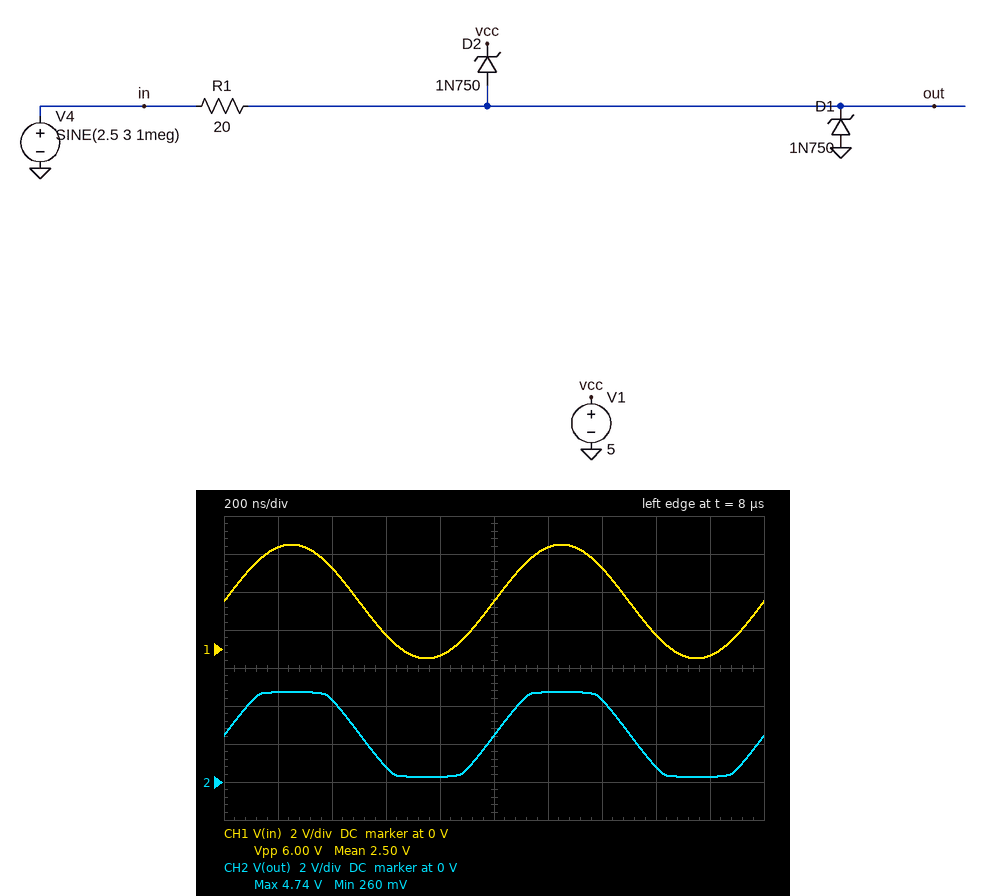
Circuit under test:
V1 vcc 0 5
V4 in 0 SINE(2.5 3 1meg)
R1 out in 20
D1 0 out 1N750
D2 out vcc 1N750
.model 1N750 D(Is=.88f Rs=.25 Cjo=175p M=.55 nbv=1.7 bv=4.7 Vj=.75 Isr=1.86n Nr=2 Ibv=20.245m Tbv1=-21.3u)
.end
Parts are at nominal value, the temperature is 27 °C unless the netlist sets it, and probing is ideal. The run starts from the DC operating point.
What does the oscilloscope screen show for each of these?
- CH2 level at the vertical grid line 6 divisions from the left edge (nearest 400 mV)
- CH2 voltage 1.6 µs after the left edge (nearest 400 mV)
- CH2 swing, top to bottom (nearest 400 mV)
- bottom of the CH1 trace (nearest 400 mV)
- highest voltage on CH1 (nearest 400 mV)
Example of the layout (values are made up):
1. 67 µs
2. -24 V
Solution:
1. 4.8 V
2. 800 mV
3. 4.4 V
4. -400 mV
5. 5.6 V
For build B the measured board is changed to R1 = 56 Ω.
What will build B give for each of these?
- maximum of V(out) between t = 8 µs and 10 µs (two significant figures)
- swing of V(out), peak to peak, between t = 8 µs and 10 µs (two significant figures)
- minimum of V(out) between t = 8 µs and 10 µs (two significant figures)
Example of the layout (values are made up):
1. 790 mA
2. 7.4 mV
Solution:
1. 4.7 V
2. 4.4 V
3. 310 mV
